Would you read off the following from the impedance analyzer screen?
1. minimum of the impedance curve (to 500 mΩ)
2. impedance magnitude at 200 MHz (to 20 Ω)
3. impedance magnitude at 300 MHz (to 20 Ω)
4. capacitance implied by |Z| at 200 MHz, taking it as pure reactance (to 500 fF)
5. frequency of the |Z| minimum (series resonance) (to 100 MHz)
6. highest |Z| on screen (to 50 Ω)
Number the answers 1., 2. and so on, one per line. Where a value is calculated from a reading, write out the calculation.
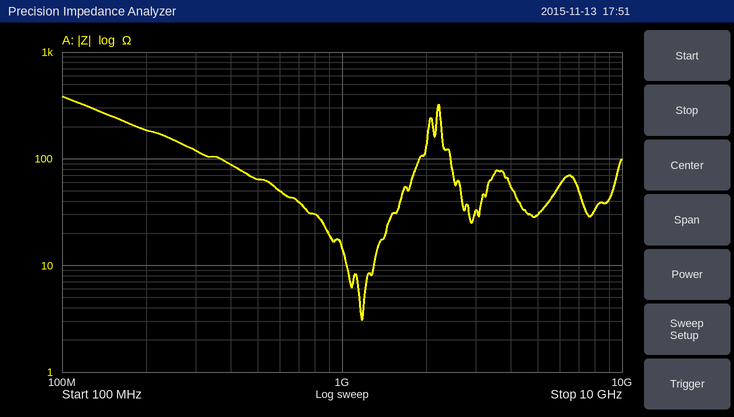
1. 3.0 Ω
2. 180 Ω
3. 120 Ω
4. C = 1/(2π × 200 MHz × 180 Ω) ≈ 4.42 pF, so 4.5 pF to the nearest 500 fF
5. 1.2 GHz
6. 400 Ω
